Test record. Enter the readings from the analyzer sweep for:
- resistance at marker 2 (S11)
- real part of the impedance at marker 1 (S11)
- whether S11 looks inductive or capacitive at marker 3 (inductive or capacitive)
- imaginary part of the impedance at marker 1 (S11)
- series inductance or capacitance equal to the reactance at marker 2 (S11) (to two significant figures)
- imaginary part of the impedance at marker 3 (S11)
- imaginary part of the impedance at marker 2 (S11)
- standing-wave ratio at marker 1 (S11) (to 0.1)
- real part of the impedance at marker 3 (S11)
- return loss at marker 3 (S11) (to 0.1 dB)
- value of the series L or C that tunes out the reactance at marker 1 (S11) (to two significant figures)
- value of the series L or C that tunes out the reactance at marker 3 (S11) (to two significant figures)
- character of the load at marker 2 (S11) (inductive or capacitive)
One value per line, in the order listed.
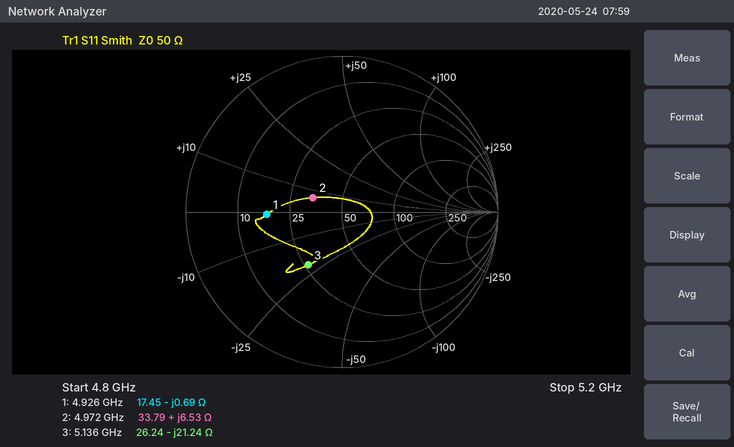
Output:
33.79 Ω
17.45 Ω
capacitive
-0.69 Ω
210 pH
-21.24 Ω
+6.53 Ω
2.9
26.24 Ω
7.9 dB
22 pH
660 pH
inductive
